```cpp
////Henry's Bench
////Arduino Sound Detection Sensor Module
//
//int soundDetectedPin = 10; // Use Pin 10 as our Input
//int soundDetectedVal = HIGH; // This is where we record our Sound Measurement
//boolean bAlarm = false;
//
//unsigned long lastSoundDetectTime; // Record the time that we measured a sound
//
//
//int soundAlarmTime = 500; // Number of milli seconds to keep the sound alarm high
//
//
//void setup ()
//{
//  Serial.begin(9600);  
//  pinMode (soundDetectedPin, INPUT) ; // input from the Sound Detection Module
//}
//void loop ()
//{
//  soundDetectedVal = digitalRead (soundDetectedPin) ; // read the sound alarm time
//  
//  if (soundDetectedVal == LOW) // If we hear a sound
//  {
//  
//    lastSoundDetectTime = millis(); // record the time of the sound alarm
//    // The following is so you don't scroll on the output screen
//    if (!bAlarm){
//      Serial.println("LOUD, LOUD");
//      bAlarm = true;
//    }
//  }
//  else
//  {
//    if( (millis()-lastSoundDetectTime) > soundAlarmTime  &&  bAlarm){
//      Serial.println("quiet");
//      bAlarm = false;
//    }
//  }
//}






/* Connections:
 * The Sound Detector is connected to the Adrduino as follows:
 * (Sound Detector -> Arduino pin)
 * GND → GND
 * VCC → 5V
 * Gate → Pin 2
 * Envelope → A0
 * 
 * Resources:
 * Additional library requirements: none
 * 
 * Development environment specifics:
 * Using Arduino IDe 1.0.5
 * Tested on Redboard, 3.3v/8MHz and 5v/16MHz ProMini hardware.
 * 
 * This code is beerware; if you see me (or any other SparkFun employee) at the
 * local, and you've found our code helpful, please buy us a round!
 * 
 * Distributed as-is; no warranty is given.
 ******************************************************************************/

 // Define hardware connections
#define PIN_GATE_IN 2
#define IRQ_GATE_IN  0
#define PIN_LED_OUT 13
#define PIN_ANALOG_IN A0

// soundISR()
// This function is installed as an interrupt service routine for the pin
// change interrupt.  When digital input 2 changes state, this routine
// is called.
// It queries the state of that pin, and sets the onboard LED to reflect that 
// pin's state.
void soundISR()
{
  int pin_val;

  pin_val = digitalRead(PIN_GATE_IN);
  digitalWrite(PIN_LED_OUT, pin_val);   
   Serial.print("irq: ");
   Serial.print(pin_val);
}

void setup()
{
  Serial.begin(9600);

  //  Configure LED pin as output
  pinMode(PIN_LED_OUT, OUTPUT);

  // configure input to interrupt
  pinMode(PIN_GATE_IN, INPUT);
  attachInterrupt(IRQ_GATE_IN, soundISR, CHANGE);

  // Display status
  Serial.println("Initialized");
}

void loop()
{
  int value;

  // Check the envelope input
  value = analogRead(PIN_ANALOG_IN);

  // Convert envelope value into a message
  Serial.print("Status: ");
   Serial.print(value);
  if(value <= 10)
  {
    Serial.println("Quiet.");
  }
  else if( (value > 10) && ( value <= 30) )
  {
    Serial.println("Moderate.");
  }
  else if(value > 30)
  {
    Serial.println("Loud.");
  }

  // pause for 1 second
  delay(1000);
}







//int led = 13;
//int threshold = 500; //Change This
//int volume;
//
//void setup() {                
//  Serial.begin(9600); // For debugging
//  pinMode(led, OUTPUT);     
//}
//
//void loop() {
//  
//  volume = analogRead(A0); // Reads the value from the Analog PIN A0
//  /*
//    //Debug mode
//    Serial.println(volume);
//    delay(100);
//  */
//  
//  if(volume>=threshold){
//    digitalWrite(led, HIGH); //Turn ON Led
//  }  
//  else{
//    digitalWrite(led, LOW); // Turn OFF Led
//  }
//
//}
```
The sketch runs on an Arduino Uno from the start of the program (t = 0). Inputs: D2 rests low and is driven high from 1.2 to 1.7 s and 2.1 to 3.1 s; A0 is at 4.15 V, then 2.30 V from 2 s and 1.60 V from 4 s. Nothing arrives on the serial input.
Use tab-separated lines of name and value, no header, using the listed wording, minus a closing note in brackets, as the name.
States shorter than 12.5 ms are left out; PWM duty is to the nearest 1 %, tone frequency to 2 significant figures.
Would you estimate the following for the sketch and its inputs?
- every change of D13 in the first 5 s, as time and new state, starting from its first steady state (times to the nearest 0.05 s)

every change of D13 in the first 5 s, as time and new state, starting from its first steady state	0 s low; 1.2 s high; 1.7 s low; 2.1 s high; 3.1 s low
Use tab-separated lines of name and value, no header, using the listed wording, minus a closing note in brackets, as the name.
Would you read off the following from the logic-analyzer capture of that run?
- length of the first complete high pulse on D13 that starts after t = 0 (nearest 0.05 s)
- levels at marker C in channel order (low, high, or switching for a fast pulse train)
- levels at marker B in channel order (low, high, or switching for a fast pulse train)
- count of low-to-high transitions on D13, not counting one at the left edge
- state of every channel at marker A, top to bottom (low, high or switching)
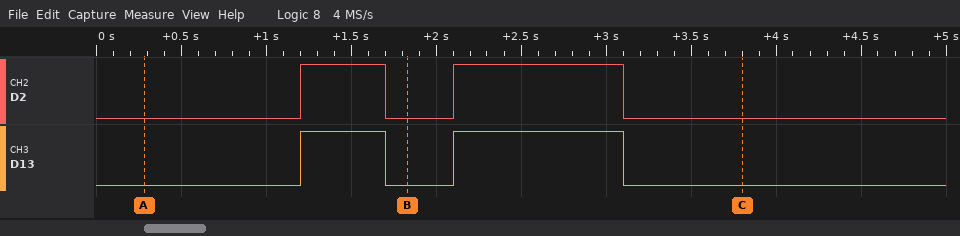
length of the first complete high pulse on D13 that starts after t = 0	0.50 s
levels at marker C in channel order	D2 low, D13 low
levels at marker B in channel order	D2 low, D13 low
count of low-to-high transitions on D13, not counting one at the left edge	2
state of every channel at marker A, top to bottom	D2 low, D13 low
